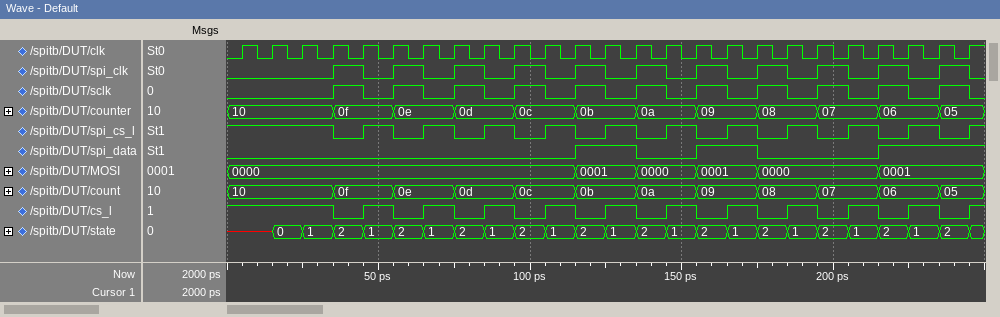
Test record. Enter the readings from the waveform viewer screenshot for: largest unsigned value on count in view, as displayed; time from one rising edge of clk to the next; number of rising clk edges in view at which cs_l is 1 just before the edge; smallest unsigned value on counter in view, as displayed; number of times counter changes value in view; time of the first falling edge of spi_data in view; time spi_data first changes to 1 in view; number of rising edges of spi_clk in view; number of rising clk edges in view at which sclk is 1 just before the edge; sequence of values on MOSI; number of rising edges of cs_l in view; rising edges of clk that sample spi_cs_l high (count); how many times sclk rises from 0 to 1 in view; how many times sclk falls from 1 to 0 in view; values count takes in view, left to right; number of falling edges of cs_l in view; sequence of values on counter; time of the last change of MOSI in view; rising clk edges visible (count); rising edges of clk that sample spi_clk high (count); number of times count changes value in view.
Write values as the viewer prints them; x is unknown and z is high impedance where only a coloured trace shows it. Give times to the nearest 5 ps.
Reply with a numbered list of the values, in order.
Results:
1. 10
2. 10 ps
3. 14
4. 05
5. 11
6. 135 ps
7. 115 ps
8. 11
9. 11
10. 0000, 0001, 0000, 0001, 0000, 0001
11. 11
12. 14
13. 11
14. 11
15. 10, 0f, 0e, 0d, 0c, 0b, 0a, 09, 08, 07, 06, 05
16. 11
17. 10, 0f, 0e, 0d, 0c, 0b, 0a, 09, 08, 07, 06, 05
18. 215 ps
19. 25
20. 11
21. 11
